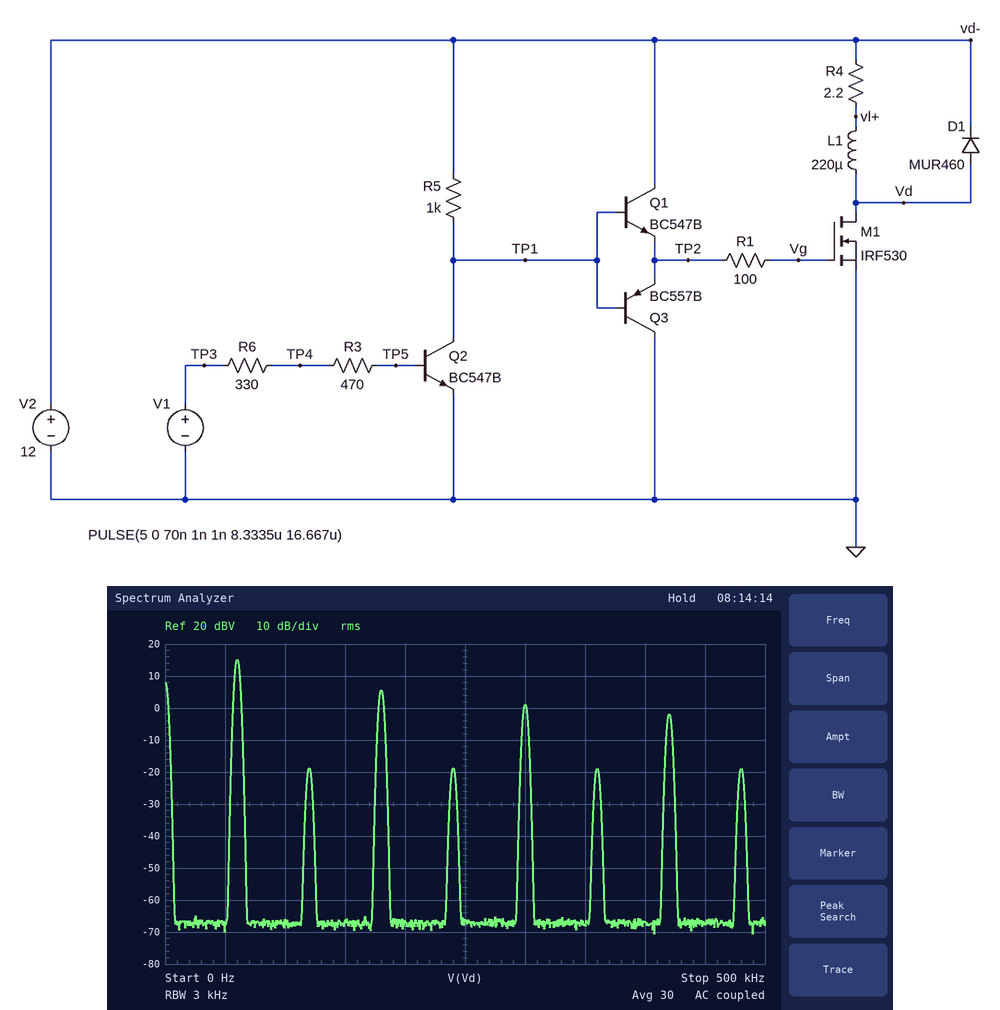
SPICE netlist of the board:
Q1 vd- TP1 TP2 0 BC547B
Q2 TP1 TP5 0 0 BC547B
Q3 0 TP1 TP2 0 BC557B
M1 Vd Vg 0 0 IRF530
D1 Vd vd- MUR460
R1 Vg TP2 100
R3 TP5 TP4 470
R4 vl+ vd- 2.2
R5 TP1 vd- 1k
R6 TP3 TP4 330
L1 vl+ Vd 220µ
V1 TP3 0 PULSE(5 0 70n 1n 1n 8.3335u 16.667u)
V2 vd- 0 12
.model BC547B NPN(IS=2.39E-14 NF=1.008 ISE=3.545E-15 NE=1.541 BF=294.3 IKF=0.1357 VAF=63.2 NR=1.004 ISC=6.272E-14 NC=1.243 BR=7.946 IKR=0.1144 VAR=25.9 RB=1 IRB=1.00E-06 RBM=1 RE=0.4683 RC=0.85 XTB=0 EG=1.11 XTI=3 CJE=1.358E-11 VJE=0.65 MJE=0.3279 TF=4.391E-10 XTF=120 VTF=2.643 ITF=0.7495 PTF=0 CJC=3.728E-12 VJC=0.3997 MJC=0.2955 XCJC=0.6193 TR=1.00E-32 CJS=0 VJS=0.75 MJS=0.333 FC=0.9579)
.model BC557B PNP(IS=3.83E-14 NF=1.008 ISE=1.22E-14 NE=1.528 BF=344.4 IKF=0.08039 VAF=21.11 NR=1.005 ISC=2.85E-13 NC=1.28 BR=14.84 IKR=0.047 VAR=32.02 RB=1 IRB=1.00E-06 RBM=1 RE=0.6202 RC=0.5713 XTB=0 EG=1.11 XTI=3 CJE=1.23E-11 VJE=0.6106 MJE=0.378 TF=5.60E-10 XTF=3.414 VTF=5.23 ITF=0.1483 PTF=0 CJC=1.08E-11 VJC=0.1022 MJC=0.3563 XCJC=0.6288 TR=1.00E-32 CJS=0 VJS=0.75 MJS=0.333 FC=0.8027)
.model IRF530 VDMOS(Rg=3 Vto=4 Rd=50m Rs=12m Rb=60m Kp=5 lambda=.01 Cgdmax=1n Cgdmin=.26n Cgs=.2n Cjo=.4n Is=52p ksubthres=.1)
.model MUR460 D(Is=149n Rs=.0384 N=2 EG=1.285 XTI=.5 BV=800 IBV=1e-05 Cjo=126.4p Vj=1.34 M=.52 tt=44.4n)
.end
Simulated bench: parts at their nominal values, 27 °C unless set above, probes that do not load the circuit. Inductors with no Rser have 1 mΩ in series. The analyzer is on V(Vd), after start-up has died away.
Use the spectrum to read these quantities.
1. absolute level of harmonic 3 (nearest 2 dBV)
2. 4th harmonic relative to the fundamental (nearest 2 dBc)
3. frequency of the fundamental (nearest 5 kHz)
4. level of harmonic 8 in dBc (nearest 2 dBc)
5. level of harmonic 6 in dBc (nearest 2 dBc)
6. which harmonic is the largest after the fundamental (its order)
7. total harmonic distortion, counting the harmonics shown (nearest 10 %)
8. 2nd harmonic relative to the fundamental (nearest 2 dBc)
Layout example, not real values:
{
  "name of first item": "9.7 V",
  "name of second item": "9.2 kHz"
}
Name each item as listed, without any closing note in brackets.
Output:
{
  "absolute level of harmonic 3": "6 dBV",
  "4th harmonic relative to the fundamental": "-34 dBc",
  "frequency of the fundamental": "60 kHz",
  "level of harmonic 8 in dBc": "-34 dBc",
  "level of harmonic 6 in dBc": "-34 dBc",
  "which harmonic is the largest after the fundamental": "3",
  "total harmonic distortion, counting the harmonics shown": "40 %",
  "2nd harmonic relative to the fundamental": "-34 dBc"
}
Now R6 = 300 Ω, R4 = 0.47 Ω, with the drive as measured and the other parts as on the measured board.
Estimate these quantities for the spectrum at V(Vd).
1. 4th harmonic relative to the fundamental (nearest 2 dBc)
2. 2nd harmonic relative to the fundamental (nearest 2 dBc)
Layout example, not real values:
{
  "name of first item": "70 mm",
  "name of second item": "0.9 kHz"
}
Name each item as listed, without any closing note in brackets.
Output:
{
  "4th harmonic relative to the fundamental": "-46 dBc",
  "2nd harmonic relative to the fundamental": "-46 dBc"
}
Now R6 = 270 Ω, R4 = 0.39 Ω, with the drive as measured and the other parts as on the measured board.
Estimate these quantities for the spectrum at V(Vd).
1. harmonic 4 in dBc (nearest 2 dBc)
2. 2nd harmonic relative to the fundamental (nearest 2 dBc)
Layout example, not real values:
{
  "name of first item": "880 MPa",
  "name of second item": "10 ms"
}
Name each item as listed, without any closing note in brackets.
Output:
{
  "harmonic 4 in dBc": "-52 dBc",
  "2nd harmonic relative to the fundamental": "-52 dBc"
}
